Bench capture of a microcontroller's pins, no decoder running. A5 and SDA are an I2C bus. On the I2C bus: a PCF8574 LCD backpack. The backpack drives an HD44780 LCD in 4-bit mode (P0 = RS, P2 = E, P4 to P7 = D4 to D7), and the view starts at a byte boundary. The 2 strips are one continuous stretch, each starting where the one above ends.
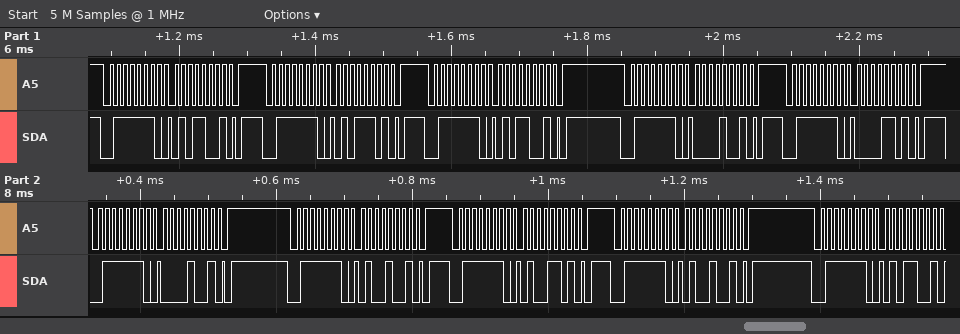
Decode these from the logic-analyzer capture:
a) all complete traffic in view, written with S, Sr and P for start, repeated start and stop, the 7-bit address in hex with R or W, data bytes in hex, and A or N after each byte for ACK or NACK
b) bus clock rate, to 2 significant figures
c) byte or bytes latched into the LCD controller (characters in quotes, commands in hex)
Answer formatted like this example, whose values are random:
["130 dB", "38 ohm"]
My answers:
["S 3FW A 59 A P S 3FW A 5D A P S 3FW A 59 A P S 3FW A 09 A P S 3FW A 0D A P S 3FW A 09 A P S 3FW A 49 A P S 3FW A 4D A P S 3FW A 49 A P S 3FW A 59 A", "100 kHz", "'P'"]
